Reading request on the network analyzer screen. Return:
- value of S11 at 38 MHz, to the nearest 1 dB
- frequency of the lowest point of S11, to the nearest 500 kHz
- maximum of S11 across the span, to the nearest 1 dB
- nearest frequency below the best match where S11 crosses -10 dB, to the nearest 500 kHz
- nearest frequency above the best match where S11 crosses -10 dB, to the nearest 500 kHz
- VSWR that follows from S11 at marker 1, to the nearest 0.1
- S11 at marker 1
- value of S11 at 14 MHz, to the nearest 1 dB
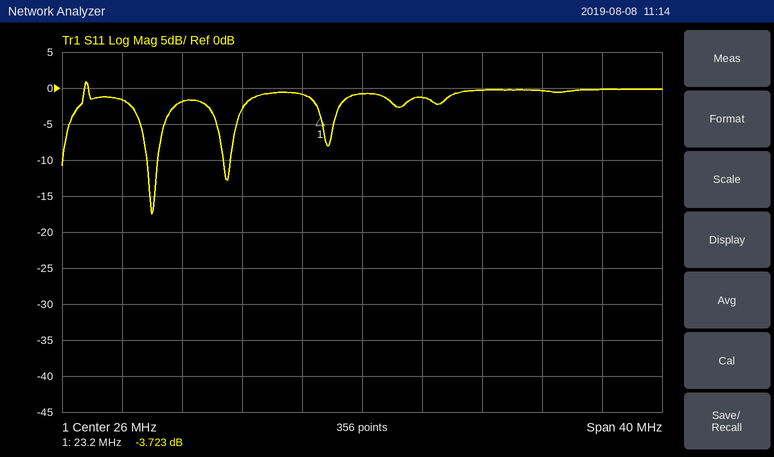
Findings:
0 dB
12.0 MHz
1 dB
11.5 MHz
12.5 MHz
4.7
-3.723 dB
-2 dB
